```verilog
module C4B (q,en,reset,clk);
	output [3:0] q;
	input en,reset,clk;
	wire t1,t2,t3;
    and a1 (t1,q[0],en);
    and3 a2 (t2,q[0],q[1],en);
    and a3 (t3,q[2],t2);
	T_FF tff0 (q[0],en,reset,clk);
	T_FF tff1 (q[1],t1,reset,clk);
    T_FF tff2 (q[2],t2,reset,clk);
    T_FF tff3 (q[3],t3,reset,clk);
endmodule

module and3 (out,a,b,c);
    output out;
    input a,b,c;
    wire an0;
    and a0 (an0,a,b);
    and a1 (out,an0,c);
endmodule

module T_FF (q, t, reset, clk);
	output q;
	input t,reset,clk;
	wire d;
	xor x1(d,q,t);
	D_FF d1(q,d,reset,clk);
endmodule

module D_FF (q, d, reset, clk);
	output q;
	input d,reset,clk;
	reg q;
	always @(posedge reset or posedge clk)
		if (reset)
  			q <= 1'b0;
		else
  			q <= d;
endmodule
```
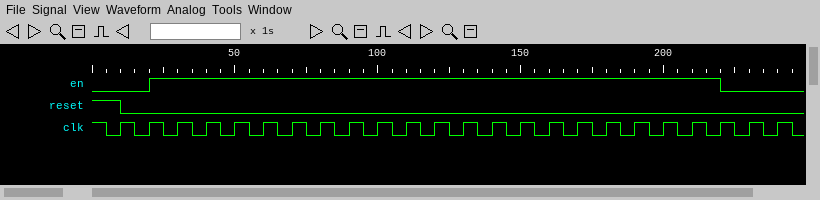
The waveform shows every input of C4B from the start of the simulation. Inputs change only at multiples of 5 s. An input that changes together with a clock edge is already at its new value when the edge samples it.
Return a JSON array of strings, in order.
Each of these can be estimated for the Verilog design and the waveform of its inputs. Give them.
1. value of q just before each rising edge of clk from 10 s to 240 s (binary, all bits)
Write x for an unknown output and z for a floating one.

["0000, 0000, 0001, 0010, 0011, 0100, 0101, 0110, 0111, 1000, 1001, 1010, 1011, 1100, 1101, 1110, 1111, 0000, 0001, 0010, 0011, 0100, 0100, 0100"]
